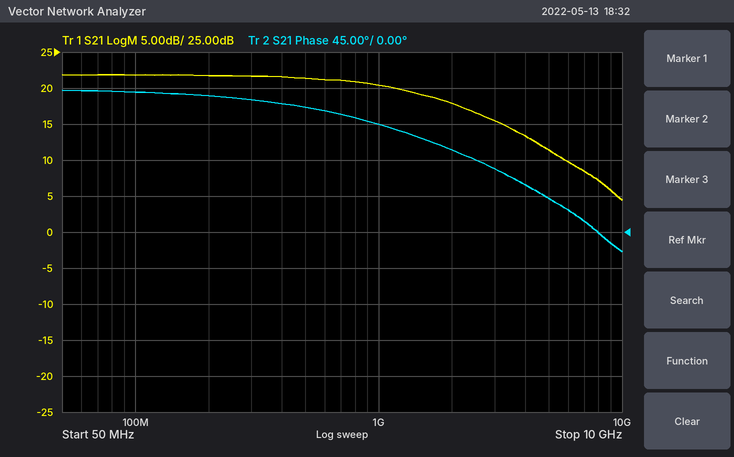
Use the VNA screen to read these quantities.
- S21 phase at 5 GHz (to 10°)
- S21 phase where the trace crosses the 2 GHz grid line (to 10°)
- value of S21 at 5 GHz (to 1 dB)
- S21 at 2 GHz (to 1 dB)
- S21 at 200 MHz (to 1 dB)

40°
100°
11 dB
18 dB
22 dB
